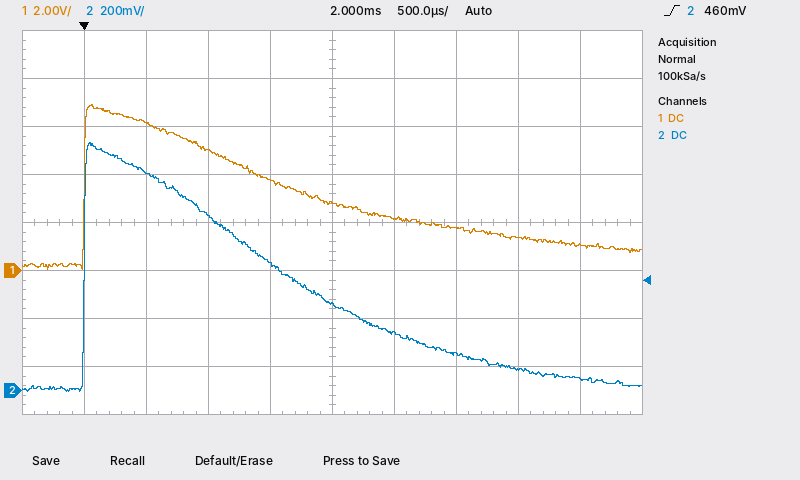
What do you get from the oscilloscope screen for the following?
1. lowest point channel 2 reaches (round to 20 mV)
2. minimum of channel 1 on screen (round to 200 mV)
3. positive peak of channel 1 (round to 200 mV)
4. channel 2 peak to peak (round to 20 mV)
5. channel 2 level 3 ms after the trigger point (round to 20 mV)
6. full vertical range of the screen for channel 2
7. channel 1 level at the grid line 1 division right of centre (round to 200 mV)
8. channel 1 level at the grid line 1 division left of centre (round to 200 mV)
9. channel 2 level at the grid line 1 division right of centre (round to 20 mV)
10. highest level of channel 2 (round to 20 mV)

0 mV
0.0 V
7.0 V
1.04 V
160 mV
1.6 V
2.2 V
3.8 V
240 mV
1.04 V
